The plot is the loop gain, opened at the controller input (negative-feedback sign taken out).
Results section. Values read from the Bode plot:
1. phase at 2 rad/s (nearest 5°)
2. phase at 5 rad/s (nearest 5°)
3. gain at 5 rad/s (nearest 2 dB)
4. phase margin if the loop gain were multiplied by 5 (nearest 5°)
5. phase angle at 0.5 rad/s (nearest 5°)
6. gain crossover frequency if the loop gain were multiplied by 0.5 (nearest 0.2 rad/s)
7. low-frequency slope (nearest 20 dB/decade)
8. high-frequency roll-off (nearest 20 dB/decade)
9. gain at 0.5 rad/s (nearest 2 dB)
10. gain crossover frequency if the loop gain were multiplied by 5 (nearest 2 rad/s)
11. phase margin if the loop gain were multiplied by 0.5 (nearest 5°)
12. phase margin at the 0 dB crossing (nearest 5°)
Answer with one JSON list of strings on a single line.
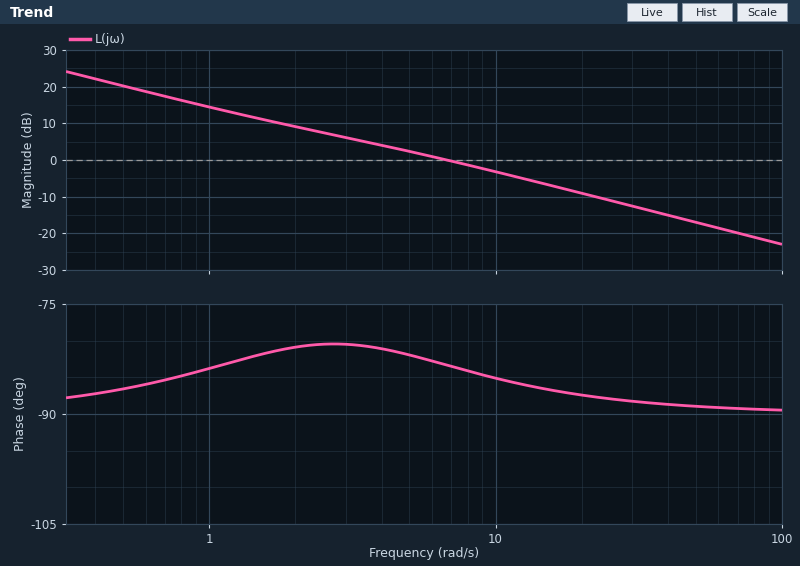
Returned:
["-80°", "-80°", "2 dB", "90°", "-85°", "3.0 rad/s", "-20 dB/decade", "-20 dB/decade", "20 dB", "36 rad/s", "100°", "95°"]
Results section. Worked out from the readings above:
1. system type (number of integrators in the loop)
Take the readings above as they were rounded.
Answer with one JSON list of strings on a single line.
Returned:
["1"]
